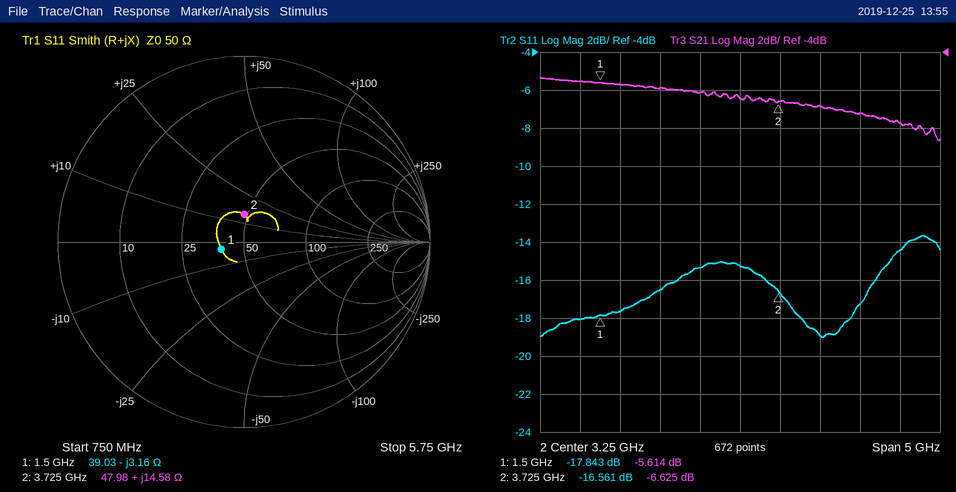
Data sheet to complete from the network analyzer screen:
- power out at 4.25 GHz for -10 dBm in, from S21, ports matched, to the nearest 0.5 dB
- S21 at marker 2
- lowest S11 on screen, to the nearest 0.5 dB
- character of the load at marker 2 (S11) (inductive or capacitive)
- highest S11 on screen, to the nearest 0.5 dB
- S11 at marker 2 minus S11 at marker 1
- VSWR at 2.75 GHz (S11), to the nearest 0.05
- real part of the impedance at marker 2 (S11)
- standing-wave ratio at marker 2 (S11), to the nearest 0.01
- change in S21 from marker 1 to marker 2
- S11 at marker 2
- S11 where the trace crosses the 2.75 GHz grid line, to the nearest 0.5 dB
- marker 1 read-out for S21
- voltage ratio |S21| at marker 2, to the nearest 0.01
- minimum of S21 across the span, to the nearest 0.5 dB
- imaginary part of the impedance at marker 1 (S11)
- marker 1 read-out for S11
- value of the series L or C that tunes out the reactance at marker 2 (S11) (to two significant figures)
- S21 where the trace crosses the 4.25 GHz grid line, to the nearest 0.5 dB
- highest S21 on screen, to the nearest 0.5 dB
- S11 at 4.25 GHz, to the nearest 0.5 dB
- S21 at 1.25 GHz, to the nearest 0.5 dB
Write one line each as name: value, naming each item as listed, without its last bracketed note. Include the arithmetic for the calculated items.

power out at 4.25 GHz for -10 dBm in, from S21, ports matched, to the nearest 0.5 dB: -10 dBm + (-7.0 dB) = -17.0 dBm
S21 at marker 2: -6.625 dB
lowest S11 on screen, to the nearest 0.5 dB: -19.0 dB
character of the load at marker 2 (S11): inductive
highest S11 on screen, to the nearest 0.5 dB: -13.5 dB
S11 at marker 2 minus S11 at marker 1: -16.561 − (-17.843) = 1.282 dB
VSWR at 2.75 GHz (S11), to the nearest 0.05: |Γ| = 10^(-15.5/20) = 0.1679; VSWR = (1 + 0.1679)/(1 − 0.1679) ≈ 1.40
real part of the impedance at marker 2: 47.98 Ω
standing-wave ratio at marker 2 (S11), to the nearest 0.01: 1.35
change in S21 from marker 1 to marker 2: -6.625 − (-5.614) = -1.011 dB
S11 at marker 2: -16.561 dB
S11 where the trace crosses the 2.75 GHz grid line, to the nearest 0.5 dB: -15.5 dB
marker 1 read-out for S21: -5.614 dB
voltage ratio |S21| at marker 2, to the nearest 0.01: 10^(-6.625/20) ≈ 0.47
minimum of S21 across the span, to the nearest 0.5 dB: -8.5 dB
imaginary part of the impedance at marker 1: -3.16 Ω
marker 1 read-out for S11: -17.843 dB
value of the series L or C that tunes out the reactance at marker 2 (S11): C = 1/(2π × 3.725 GHz × 14.58 Ω) ≈ 2.9 pF
S21 where the trace crosses the 4.25 GHz grid line, to the nearest 0.5 dB: -7.0 dB
highest S21 on screen, to the nearest 0.5 dB: -5.5 dB
S11 at 4.25 GHz, to the nearest 0.5 dB: -19.0 dB
S21 at 1.25 GHz, to the nearest 0.5 dB: -5.5 dB
